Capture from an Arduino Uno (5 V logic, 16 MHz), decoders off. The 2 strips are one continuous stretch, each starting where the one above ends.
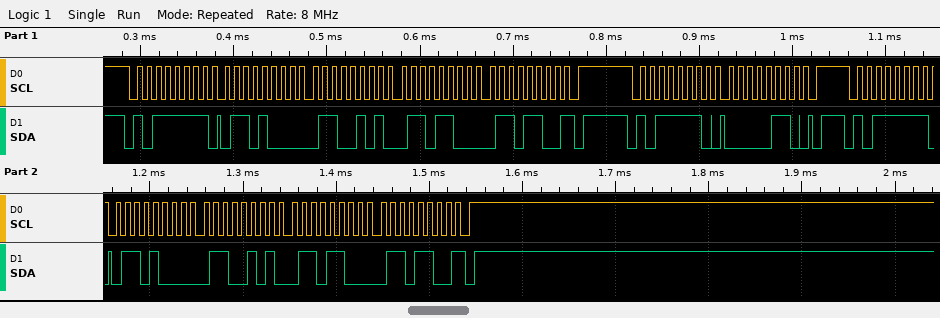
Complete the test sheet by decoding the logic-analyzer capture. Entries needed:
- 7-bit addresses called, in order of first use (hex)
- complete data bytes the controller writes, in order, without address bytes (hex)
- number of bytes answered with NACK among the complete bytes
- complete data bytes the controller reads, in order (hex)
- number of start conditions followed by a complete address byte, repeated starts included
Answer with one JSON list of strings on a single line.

["0x5F", "06", "2", "68 65 6C 6C 68 65 6C 6C", "3"]
